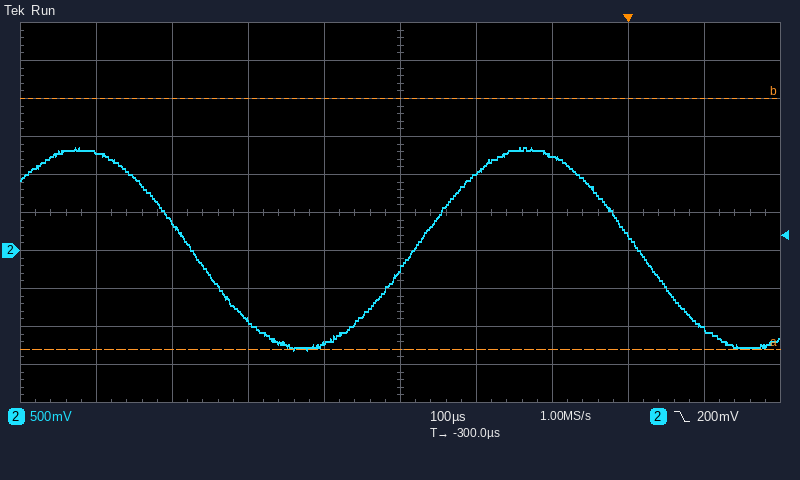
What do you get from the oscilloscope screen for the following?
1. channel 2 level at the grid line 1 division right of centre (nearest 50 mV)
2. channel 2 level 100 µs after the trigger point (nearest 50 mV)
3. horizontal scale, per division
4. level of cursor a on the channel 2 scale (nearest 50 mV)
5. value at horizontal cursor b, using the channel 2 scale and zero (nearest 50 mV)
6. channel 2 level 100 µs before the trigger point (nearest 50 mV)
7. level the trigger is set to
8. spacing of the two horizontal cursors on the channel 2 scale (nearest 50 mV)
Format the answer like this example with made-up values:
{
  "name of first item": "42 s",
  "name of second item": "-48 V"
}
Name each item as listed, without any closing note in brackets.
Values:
{
  "channel 2 level at the grid line 1 division right of centre": "1.00 V",
  "channel 2 level 100 µs after the trigger point": "-1.05 V",
  "horizontal scale, per division": "100 µs",
  "level of cursor a on the channel 2 scale": "-1.30 V",
  "value at horizontal cursor b, using the channel 2 scale and zero": "2.00 V",
  "channel 2 level 100 µs before the trigger point": "1.25 V",
  "level the trigger is set to": "200 mV",
  "spacing of the two horizontal cursors on the channel 2 scale": "3.30 V"
}
